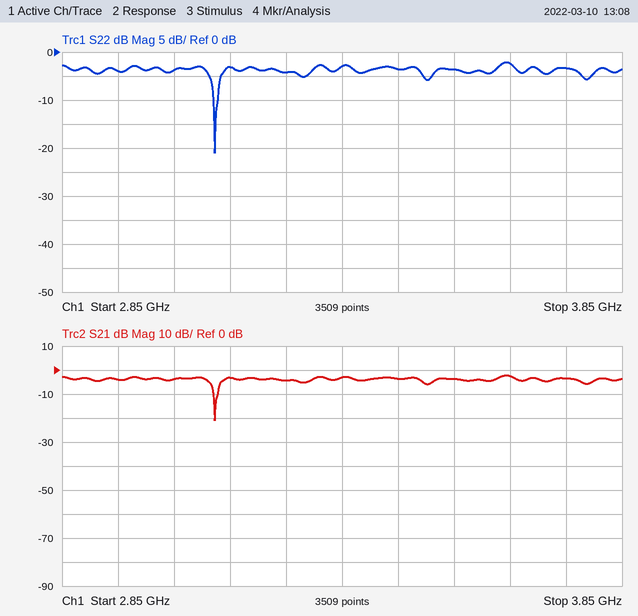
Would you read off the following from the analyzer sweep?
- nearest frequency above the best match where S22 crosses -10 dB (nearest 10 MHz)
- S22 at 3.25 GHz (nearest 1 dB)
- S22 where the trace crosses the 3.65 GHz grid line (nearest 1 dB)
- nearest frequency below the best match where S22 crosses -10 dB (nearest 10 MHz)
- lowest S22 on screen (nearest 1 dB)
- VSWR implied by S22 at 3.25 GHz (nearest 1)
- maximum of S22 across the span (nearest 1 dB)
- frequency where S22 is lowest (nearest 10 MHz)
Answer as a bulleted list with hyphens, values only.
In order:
- 3.13 GHz
- -4 dB
- -2 dB
- 3.12 GHz
- -21 dB
- 4
- -2 dB
- 3.12 GHz
